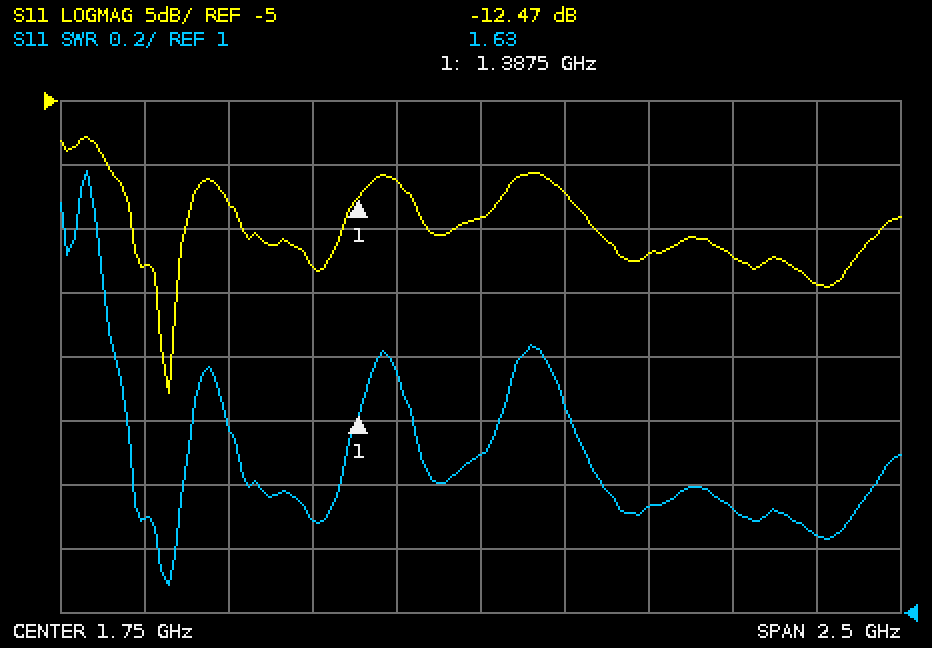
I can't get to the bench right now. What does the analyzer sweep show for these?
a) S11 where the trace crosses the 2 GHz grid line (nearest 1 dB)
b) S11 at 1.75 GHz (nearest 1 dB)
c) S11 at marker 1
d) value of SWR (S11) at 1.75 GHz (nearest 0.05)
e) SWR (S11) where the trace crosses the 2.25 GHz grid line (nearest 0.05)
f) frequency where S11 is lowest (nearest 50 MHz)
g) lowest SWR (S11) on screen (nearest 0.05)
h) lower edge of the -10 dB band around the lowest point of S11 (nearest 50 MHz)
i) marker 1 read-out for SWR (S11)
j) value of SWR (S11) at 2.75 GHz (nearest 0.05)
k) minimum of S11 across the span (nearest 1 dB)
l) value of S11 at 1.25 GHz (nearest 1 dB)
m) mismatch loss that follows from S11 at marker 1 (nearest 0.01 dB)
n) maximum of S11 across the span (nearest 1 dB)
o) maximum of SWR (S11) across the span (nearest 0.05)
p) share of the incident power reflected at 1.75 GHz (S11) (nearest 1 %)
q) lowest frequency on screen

-12 dB
-14 dB
-12.47 dB
1.50
1.35
800 MHz
1.10
650 MHz
1.63
1.25
-28 dB
-18 dB
0.25 dB
-8 dB
2.40
4 %
500 MHz
